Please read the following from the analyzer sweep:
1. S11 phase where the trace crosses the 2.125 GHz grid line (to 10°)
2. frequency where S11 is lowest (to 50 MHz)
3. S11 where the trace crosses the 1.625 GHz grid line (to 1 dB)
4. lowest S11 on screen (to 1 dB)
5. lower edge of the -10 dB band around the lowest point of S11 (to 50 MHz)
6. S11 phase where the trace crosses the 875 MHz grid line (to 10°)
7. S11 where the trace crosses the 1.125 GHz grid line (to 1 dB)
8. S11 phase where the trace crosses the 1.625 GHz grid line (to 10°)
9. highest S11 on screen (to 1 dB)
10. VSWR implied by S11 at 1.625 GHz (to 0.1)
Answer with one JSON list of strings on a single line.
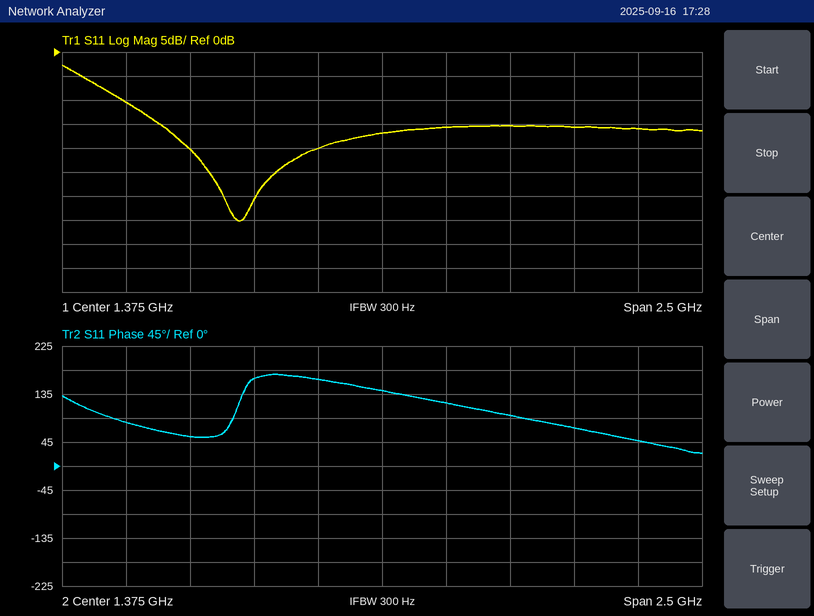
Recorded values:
["70°", "800 MHz", "-16 dB", "-35 dB", "350 MHz", "160°", "-20 dB", "120°", "-3 dB", "1.4"]
